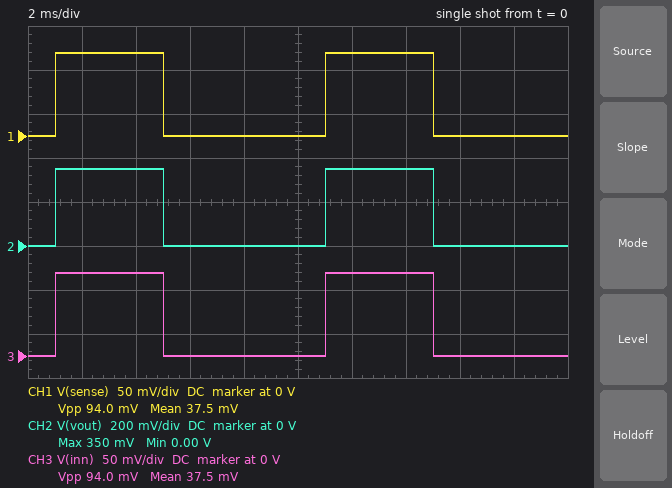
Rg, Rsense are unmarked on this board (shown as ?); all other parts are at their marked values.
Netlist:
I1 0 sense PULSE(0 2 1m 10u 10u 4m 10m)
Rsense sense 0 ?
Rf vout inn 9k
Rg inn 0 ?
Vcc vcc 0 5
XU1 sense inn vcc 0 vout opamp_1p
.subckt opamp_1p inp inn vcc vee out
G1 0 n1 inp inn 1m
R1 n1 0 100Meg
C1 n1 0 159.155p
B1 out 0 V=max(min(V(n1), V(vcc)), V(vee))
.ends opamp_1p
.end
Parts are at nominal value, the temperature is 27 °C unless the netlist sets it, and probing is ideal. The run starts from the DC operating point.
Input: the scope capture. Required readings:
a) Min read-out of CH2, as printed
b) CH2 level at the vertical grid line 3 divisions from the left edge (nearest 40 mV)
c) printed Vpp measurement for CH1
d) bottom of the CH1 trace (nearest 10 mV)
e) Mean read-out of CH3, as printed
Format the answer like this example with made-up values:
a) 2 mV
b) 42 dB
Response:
a) 0.00 V
b) 0 V
c) 94.0 mV
d) 0 V
e) 37.5 mV
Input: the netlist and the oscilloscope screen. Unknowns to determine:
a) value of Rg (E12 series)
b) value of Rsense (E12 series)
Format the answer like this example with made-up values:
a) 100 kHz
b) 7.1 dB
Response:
a) 3.3 kΩ
b) 0.047 Ω
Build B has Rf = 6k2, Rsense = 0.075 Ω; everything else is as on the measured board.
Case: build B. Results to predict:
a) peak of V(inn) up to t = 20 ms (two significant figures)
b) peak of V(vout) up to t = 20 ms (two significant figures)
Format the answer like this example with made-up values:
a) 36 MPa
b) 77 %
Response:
a) 150 mV
b) 430 mV
